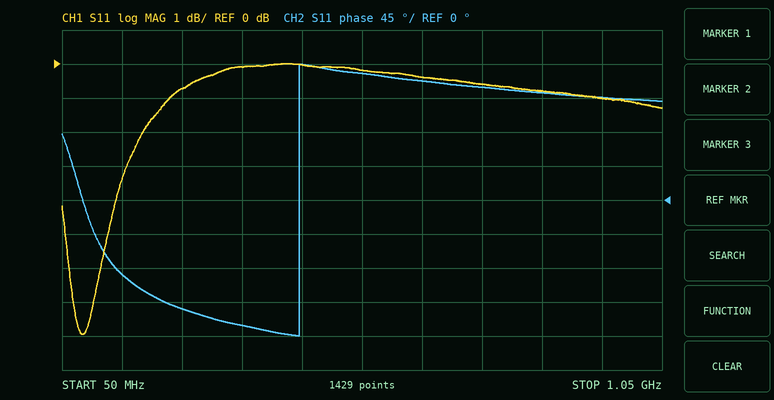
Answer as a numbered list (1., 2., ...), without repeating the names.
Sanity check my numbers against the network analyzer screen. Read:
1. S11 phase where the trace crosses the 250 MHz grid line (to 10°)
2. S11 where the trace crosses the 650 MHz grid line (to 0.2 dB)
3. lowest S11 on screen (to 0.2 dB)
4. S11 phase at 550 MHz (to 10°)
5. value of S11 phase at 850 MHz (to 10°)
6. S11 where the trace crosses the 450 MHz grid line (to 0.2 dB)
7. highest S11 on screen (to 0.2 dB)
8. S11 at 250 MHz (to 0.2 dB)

1. -140°
2. -0.4 dB
3. -8.0 dB
4. 170°
5. 140°
6. 0.0 dB
7. 0.0 dB
8. -0.8 dB
